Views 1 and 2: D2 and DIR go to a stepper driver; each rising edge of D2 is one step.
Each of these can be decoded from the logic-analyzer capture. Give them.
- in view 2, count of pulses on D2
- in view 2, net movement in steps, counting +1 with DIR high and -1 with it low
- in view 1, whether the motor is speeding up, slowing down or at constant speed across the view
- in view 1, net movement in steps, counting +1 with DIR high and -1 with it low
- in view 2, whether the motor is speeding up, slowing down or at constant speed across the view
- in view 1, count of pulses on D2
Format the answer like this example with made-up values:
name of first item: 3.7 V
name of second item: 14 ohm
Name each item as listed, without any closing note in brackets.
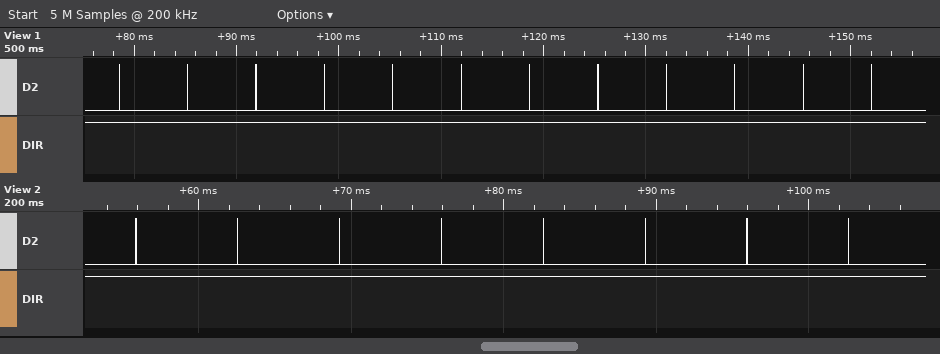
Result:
in view 2, count of pulses on D2: 8
in view 2, net movement in steps, counting +1 with DIR high and -1 with it low: +8
in view 1, whether the motor is speeding up, slowing down or at constant speed across the view: constant speed
in view 1, net movement in steps, counting +1 with DIR high and -1 with it low: +12
in view 2, whether the motor is speeding up, slowing down or at constant speed across the view: constant speed
in view 1, count of pulses on D2: 12
